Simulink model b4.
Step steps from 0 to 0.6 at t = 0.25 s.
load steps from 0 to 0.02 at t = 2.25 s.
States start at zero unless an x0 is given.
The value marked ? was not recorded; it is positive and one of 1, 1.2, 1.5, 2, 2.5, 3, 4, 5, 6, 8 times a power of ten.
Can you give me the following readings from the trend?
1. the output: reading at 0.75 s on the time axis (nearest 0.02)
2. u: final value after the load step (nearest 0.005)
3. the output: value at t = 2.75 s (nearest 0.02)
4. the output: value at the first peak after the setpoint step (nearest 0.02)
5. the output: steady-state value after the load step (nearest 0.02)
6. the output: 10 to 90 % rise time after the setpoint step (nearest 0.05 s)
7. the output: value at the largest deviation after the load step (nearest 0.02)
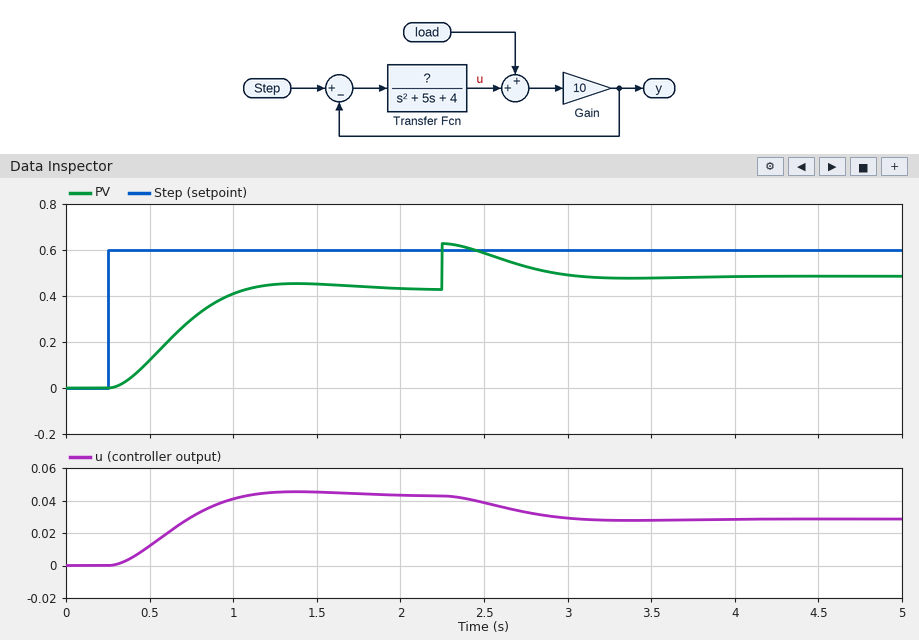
0.30
0.030
0.52
0.46
0.48
0.55 s
0.62
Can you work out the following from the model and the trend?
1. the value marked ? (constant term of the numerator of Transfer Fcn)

1
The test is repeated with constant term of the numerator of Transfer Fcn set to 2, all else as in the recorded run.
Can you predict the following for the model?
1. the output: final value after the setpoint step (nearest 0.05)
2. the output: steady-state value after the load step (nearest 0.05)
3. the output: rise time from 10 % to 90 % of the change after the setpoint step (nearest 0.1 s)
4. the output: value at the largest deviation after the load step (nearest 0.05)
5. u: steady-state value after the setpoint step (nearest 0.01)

0.50
0.55
0.3 s
0.70
0.05
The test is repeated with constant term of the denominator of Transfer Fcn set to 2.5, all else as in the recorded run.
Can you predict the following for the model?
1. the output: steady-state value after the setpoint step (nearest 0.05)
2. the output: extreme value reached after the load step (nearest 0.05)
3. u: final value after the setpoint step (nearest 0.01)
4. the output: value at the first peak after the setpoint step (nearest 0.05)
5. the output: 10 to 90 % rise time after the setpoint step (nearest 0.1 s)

0.50
0.70
0.05
0.50
0.6 s
